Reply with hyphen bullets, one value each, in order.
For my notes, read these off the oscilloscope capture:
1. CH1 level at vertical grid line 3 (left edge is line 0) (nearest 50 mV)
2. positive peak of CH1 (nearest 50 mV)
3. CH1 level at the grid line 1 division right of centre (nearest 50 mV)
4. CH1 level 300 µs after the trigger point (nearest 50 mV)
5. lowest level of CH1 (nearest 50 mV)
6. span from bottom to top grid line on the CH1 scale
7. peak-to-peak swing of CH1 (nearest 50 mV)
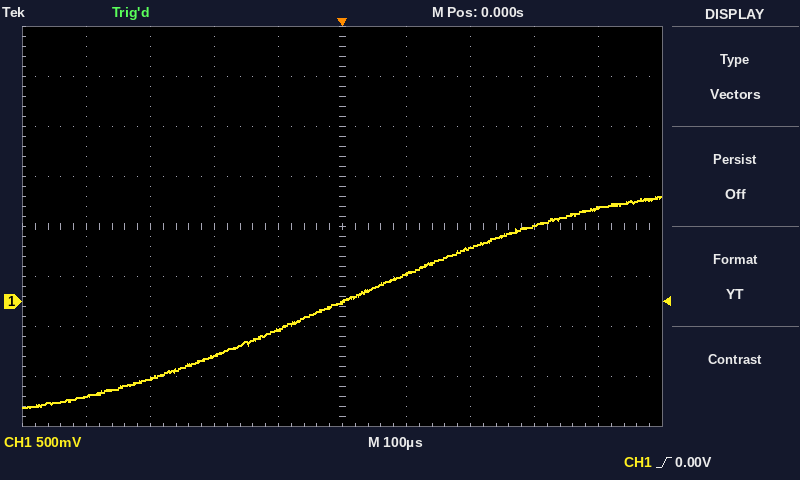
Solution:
- -550 mV
- 1.05 V
- 300 mV
- 750 mV
- -1.05 V
- 4 V
- 2.10 V
